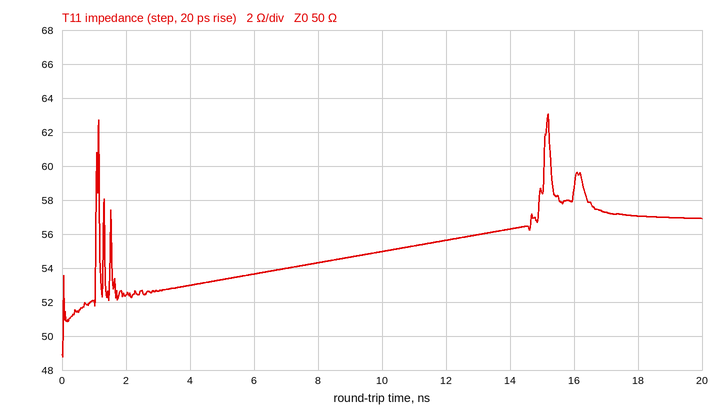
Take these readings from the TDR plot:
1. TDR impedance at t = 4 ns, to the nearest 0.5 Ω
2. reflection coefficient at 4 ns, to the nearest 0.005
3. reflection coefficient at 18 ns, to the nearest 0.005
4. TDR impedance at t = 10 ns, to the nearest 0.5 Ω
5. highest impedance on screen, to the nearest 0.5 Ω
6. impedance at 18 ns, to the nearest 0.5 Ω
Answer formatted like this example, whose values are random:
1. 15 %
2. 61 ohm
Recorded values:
1. 53.0 Ω
2. +0.030
3. +0.065
4. 55.0 Ω
5. 63.0 Ω
6. 57.0 Ω
